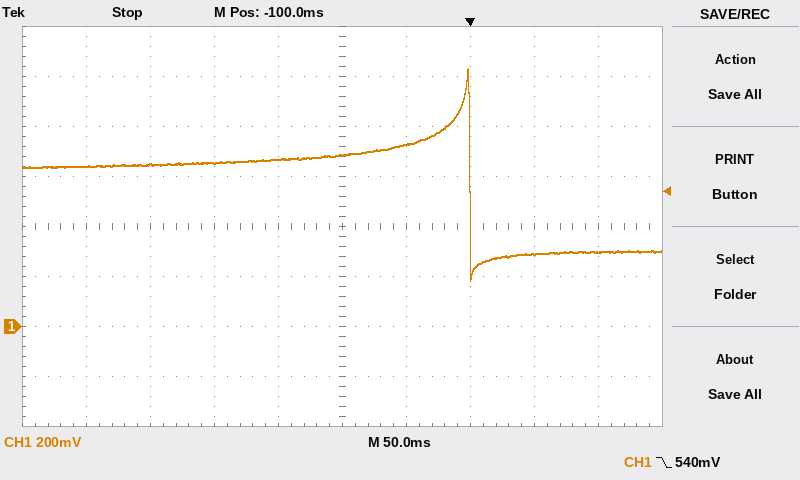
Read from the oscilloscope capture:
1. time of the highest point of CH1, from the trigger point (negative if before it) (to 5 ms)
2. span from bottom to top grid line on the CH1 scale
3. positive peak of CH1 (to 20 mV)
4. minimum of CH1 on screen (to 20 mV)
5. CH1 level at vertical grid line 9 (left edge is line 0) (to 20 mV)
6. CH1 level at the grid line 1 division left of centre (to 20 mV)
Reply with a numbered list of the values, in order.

1. 0 ms
2. 1.6 V
3. 1.04 V
4. 180 mV
5. 300 mV
6. 660 mV
